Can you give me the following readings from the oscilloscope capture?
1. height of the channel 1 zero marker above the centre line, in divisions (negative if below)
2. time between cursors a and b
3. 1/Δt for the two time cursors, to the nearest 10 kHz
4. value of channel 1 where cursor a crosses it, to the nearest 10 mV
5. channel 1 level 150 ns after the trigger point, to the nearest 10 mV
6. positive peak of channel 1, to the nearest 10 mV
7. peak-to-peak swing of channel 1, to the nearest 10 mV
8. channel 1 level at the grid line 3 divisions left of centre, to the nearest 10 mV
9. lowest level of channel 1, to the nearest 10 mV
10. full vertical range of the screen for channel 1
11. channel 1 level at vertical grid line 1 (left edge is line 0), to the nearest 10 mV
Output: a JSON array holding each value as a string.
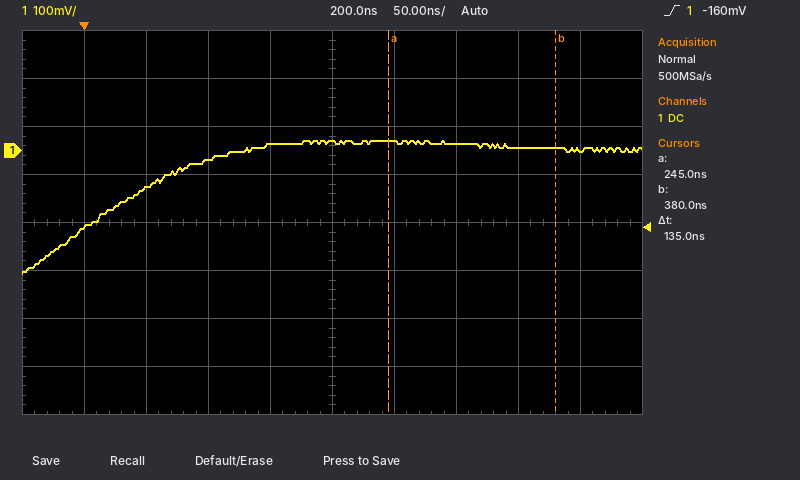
["+1.5 div", "135 ns", "7.41 MHz", "20 mV", "10 mV", "20 mV", "280 mV", "-80 mV", "-260 mV", "800 mV", "-160 mV"]
